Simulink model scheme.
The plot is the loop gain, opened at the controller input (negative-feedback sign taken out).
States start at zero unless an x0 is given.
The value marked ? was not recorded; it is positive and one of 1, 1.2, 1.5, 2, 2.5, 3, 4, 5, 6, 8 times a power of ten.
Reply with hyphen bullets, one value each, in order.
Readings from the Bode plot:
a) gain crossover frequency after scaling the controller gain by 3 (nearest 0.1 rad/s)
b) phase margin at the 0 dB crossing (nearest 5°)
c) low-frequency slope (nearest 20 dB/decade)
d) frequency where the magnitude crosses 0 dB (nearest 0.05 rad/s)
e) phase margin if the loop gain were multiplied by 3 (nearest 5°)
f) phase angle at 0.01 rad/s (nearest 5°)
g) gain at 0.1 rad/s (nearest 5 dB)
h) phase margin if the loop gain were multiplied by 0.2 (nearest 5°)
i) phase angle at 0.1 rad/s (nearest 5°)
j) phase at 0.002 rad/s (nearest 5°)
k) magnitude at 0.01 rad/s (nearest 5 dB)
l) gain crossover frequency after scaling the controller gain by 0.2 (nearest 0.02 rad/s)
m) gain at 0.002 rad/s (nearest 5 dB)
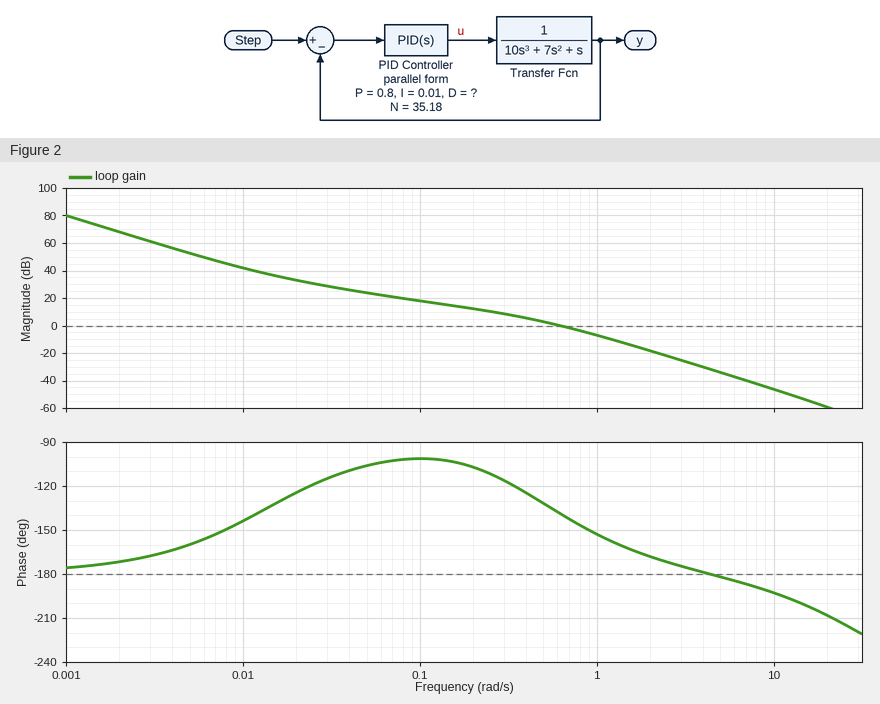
- 1.2 rad/s
- 40°
- -40 dB/decade
- 0.60 rad/s
- 25°
- -145°
- 20 dB
- 75°
- -100°
- -170°
- 40 dB
- 0.16 rad/s
- 70 dB
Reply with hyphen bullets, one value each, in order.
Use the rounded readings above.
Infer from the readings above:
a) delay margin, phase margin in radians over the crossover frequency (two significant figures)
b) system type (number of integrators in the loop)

- 1.2 s
- 2
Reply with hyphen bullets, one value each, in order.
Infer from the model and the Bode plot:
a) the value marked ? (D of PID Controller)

- 5
